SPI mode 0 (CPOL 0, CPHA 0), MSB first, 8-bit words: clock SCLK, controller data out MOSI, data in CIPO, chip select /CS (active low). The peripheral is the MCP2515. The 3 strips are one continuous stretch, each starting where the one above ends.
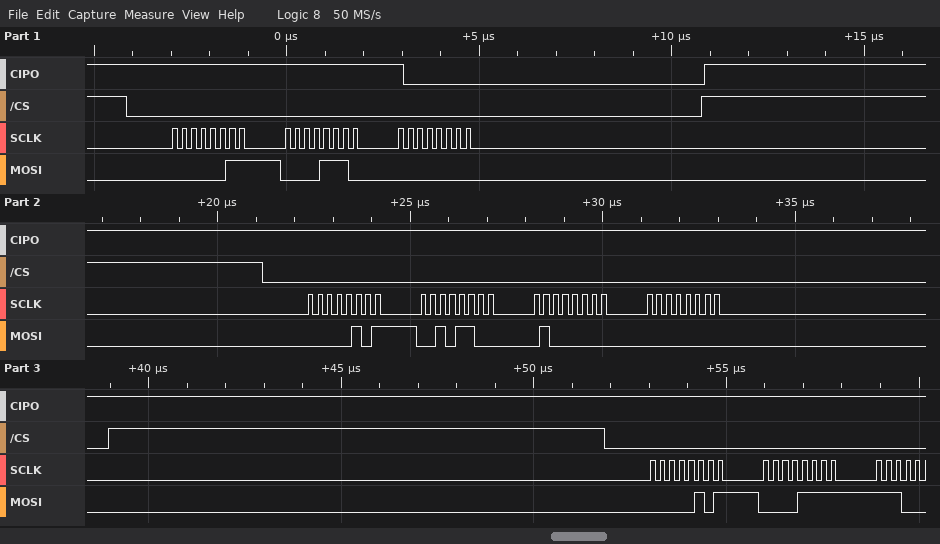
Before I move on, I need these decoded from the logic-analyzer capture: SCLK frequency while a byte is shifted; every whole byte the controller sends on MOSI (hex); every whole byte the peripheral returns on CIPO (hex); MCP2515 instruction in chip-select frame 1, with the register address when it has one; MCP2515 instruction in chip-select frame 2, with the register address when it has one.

4 MHz
03 0E 00 05 2C 40 00 05 0F
FF FF 80 FF FF FF FF FF FF
READ 0x0E
BIT MODIFY 0x2C
